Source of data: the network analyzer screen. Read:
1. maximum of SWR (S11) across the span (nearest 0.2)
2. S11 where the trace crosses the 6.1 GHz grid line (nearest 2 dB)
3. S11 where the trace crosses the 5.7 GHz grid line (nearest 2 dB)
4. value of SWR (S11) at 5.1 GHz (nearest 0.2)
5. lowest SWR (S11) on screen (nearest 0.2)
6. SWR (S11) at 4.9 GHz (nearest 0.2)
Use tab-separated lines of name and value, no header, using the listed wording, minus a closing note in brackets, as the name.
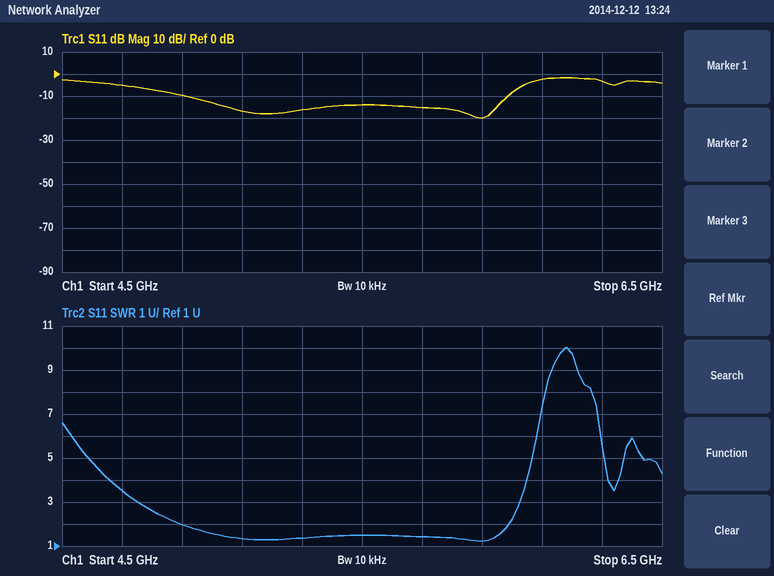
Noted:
maximum of SWR (S11) across the span	10.0
S11 where the trace crosses the 6.1 GHz grid line	-2 dB
S11 where the trace crosses the 5.7 GHz grid line	-16 dB
value of SWR (S11) at 5.1 GHz	1.4
lowest SWR (S11) on screen	1.2
SWR (S11) at 4.9 GHz	2.0
